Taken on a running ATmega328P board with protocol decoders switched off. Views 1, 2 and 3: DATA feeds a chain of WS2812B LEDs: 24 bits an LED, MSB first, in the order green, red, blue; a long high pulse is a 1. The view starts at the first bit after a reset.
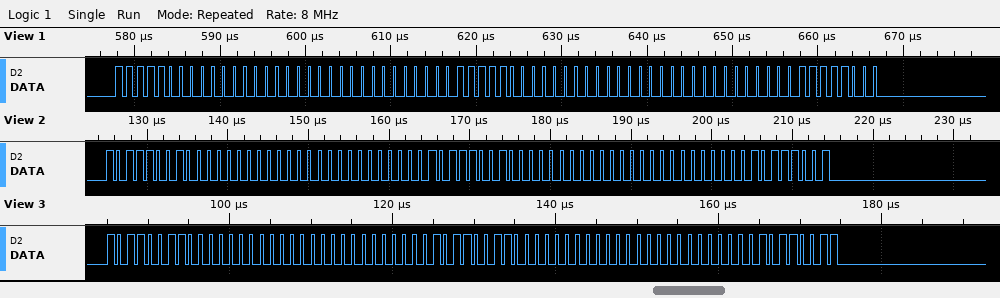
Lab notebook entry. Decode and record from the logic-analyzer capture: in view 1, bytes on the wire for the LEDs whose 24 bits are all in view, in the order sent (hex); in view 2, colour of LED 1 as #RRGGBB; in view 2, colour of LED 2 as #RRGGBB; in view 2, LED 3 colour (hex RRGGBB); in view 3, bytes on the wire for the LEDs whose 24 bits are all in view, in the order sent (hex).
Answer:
F8 00 00 00 F8 00 00 00 F8
#00B900
#B90000
#0000B9
B3 00 00 00 B3 00 00 00 B3
